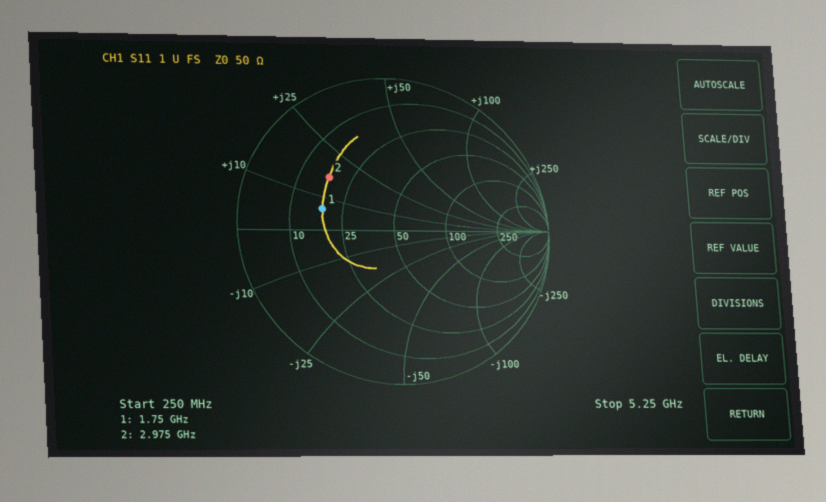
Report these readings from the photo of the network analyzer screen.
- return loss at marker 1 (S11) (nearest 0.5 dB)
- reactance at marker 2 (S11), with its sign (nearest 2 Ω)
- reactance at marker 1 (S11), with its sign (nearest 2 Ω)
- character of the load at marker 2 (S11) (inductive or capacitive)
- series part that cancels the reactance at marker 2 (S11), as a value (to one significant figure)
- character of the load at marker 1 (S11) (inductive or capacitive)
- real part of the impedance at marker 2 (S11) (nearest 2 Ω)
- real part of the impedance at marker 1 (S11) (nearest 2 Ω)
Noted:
6.5 dB
+16 Ω
+6 Ω
inductive
3 pF
inductive
18 Ω
18 Ω
